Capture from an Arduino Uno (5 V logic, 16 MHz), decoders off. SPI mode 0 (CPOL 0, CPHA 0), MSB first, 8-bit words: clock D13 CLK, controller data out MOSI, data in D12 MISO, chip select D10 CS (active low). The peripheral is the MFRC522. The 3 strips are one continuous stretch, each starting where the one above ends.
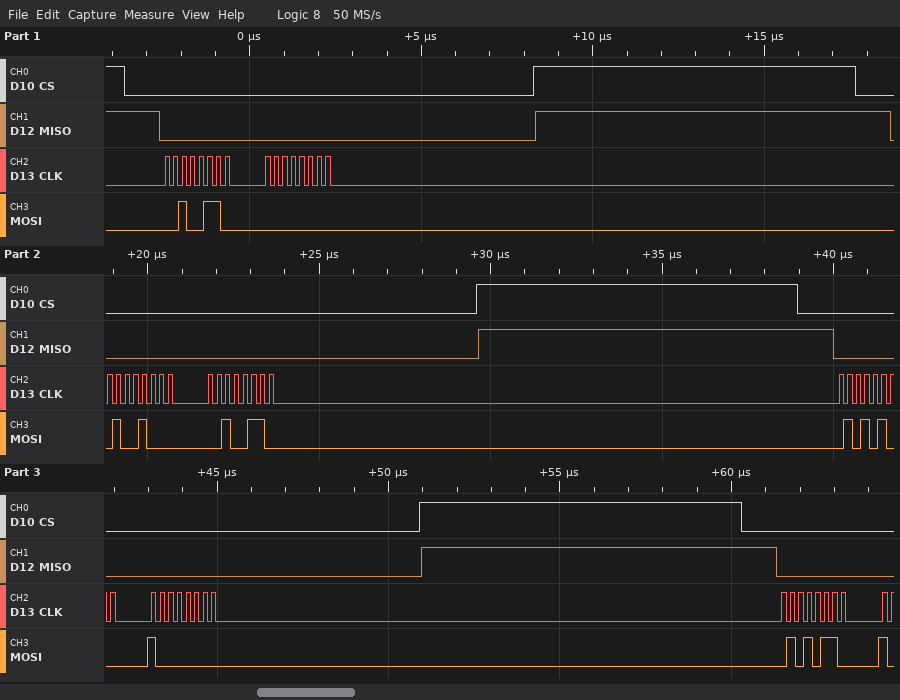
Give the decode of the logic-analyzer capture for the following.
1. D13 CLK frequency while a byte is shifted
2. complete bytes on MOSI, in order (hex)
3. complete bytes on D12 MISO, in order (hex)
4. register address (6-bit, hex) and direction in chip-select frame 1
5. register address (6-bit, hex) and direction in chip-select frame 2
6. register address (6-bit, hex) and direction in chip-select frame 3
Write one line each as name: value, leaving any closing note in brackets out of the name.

D13 CLK frequency while a byte is shifted: 4 MHz
complete bytes on MOSI, in order: 26 00 48 26 54 80 56
complete bytes on D12 MISO, in order: 00 00 00 00 00 00 00
register address (6-bit, hex) and direction in chip-select frame 1: 0x13 write
register address (6-bit, hex) and direction in chip-select frame 2: 0x24 write
register address (6-bit, hex) and direction in chip-select frame 3: 0x2A write
